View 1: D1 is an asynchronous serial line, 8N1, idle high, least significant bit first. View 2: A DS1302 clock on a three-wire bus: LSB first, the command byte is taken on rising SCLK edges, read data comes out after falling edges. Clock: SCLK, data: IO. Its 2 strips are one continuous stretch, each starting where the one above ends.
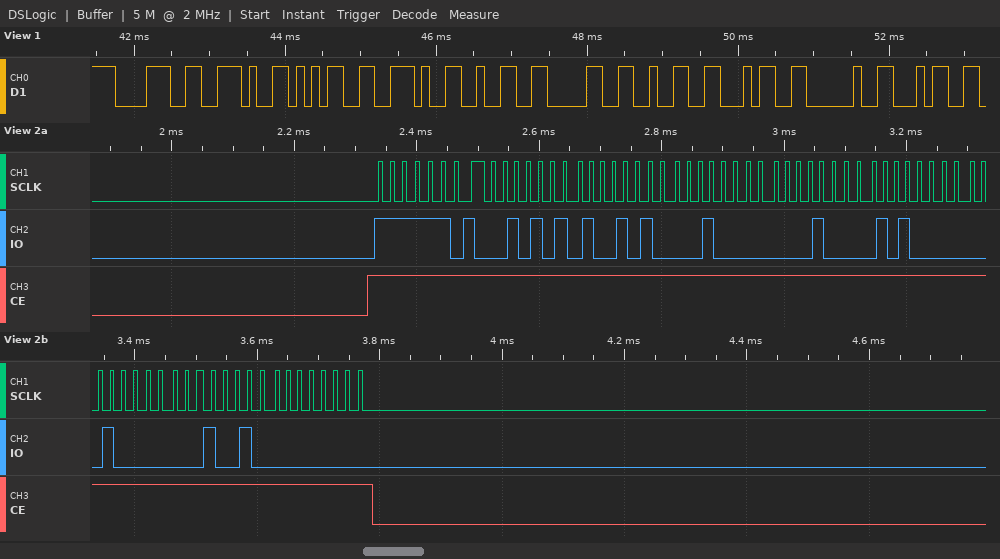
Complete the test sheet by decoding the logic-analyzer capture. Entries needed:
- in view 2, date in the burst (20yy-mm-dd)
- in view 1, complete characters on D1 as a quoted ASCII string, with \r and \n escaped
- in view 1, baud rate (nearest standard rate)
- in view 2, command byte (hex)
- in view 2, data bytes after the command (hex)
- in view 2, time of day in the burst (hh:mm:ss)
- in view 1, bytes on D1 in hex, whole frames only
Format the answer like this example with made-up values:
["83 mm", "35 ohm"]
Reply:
["2024-05-08", "\"8.5.2024 4\"", "9600 baud", "0xBF", "54 29 04 08 05 04 24 00", "04:29:54", "38 2E 35 2E 32 30 32 34 20 34"]
